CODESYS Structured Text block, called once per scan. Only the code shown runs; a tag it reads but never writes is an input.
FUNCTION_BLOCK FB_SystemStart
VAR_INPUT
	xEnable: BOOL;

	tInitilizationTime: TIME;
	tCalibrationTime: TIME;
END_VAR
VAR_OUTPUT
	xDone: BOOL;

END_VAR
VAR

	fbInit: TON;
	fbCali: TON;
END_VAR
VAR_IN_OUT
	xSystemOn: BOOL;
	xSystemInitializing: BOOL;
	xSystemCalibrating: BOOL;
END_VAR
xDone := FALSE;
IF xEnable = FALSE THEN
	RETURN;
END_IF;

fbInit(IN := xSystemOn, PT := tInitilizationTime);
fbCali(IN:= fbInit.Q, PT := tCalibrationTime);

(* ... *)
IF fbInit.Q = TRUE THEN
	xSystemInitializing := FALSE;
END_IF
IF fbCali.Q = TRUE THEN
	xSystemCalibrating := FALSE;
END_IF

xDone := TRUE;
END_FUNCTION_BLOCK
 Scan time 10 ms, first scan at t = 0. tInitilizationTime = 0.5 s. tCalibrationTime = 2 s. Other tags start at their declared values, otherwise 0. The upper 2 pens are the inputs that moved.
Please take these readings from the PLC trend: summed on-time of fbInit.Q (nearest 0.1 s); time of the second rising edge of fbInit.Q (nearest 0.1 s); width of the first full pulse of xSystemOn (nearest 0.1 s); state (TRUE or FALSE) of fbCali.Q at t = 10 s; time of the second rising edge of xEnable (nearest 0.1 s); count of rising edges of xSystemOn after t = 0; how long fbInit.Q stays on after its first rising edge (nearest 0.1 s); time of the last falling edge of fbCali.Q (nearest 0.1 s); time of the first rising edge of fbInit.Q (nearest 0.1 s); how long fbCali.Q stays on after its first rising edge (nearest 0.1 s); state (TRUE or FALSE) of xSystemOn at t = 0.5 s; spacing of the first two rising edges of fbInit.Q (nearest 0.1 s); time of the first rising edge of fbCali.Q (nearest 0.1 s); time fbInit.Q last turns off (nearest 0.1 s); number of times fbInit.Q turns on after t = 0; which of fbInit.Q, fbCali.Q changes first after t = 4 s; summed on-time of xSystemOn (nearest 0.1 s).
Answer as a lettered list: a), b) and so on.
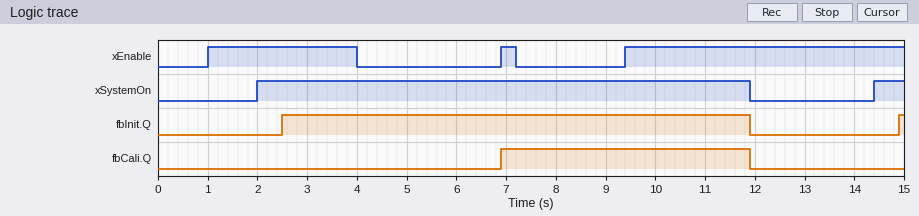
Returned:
a) 9.5 s
b) 14.9 s
c) 9.9 s
d) TRUE
e) 6.9 s
f) 2
g) 9.4 s
h) 11.9 s
i) 2.5 s
j) 5.0 s
k) FALSE
l) 12.4 s
m) 6.9 s
n) 11.9 s
o) 2
p) fbCali.Q
q) 10.5 s
